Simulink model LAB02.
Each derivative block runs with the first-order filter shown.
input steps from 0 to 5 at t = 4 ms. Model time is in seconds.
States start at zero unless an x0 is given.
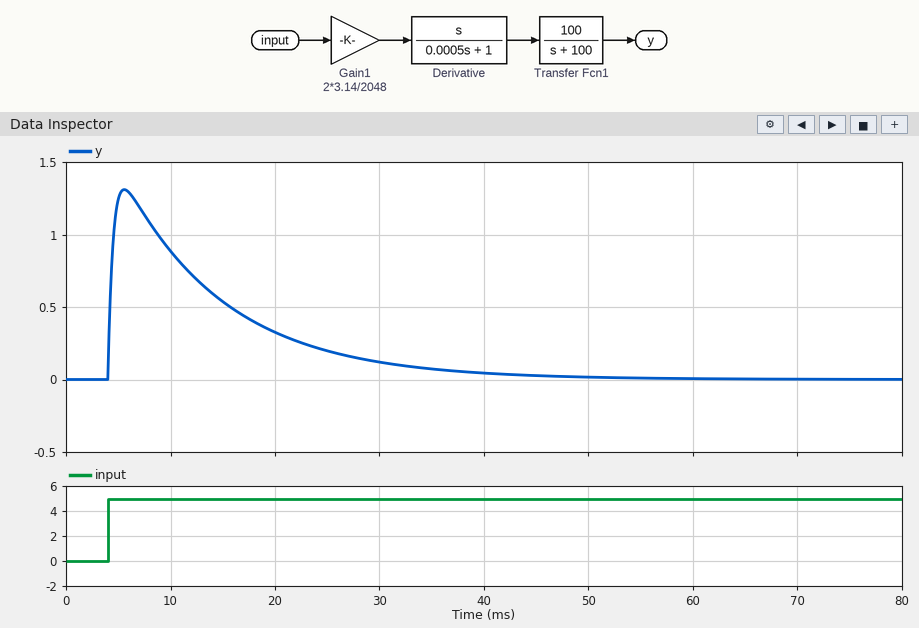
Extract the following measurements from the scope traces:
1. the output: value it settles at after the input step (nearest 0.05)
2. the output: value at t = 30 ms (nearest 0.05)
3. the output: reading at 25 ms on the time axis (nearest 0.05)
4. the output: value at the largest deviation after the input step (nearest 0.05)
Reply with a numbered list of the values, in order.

1. 0.00
2. 0.10
3. 0.20
4. 1.30
